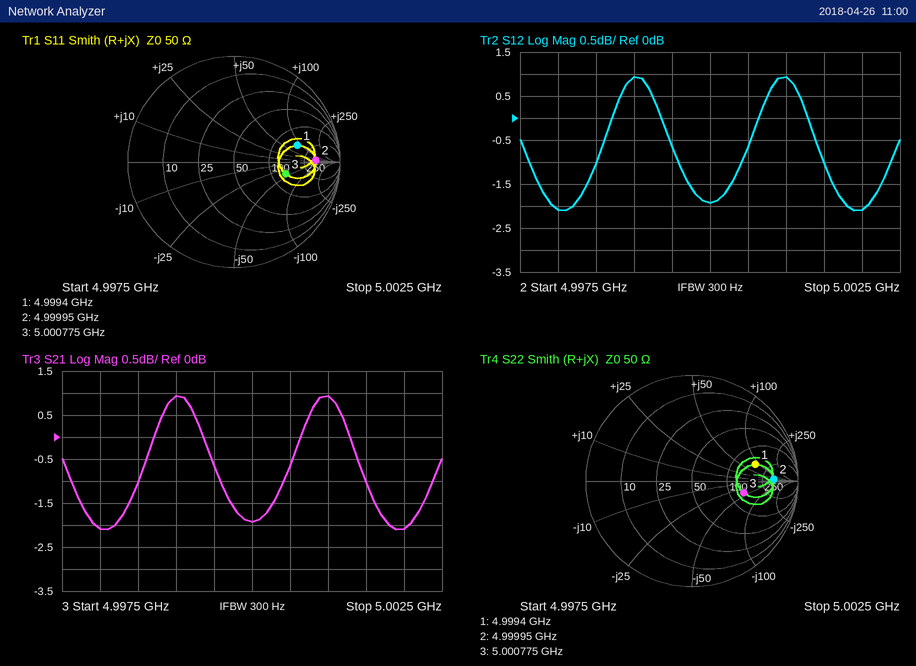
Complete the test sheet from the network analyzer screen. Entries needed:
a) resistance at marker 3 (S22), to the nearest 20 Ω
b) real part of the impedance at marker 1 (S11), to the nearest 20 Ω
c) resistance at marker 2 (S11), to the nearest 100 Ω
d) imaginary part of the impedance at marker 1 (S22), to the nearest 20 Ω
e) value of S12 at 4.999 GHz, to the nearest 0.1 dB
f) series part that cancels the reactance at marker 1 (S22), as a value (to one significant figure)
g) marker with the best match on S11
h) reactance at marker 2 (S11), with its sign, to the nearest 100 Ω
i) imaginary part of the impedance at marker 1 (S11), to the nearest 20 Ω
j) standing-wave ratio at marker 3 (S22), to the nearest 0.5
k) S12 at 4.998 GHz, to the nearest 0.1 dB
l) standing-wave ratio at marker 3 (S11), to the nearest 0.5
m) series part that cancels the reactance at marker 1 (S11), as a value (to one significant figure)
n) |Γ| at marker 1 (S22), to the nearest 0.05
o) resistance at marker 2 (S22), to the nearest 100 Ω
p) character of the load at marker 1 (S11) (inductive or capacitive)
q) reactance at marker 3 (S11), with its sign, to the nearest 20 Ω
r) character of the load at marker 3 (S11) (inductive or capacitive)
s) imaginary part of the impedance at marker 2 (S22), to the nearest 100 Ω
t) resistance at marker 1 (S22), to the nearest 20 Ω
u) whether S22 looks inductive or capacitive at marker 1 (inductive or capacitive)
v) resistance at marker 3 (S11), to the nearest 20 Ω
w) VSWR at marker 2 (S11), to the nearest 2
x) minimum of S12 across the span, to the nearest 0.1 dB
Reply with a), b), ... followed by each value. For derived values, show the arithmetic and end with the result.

a) 140 Ω
b) 160 Ω
c) 400 Ω
d) +80 Ω
e) 0.9 dB
f) C = 1/(2π × 4.9994 GHz × 80 Ω) ≈ 398 fF, so 400 fF to one significant figure
g) marker 3
h) 0 Ω
i) +80 Ω
j) 3.0
k) -2.1 dB
l) 3.0
m) C = 1/(2π × 4.9994 GHz × 80 Ω) ≈ 398 fF, so 400 fF to one significant figure
n) 0.60
o) 400 Ω
p) inductive
q) -40 Ω
r) capacitive
s) 0 Ω
t) 160 Ω
u) inductive
v) 140 Ω
w) 8
x) -2.1 dB
